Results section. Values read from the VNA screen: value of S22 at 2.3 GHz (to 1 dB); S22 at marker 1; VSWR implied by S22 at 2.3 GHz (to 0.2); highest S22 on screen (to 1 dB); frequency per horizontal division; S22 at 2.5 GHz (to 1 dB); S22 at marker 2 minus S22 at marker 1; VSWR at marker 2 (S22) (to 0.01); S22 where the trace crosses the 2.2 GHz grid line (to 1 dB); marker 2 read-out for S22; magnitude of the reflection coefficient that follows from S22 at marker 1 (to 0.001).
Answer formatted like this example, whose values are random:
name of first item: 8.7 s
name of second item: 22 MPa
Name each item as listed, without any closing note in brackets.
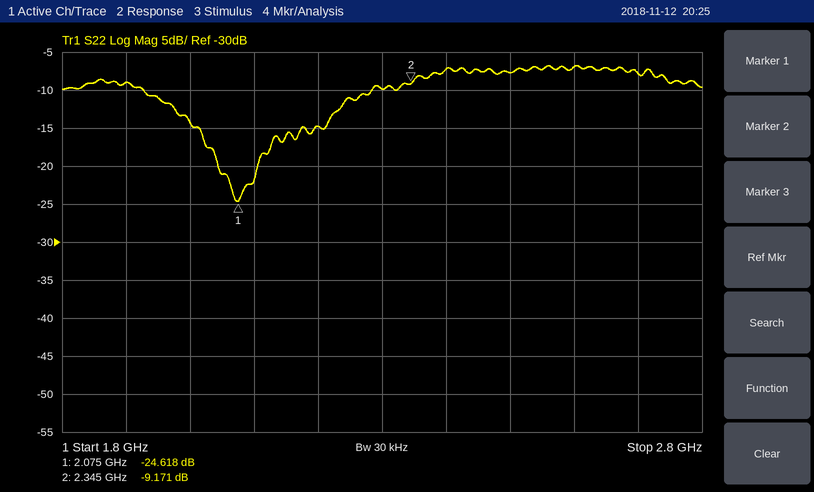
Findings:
value of S22 at 2.3 GHz: -10 dB
S22 at marker 1: -24.618 dB
VSWR implied by S22 at 2.3 GHz: 2.0
highest S22 on screen: -7 dB
frequency per horizontal division: 100 MHz
S22 at 2.5 GHz: -8 dB
S22 at marker 2 minus S22 at marker 1: 15.447 dB
VSWR at marker 2 (S22): 2.07
S22 where the trace crosses the 2.2 GHz grid line: -15 dB
marker 2 read-out for S22: -9.171 dB
magnitude of the reflection coefficient that follows from S22 at marker 1: 0.059
